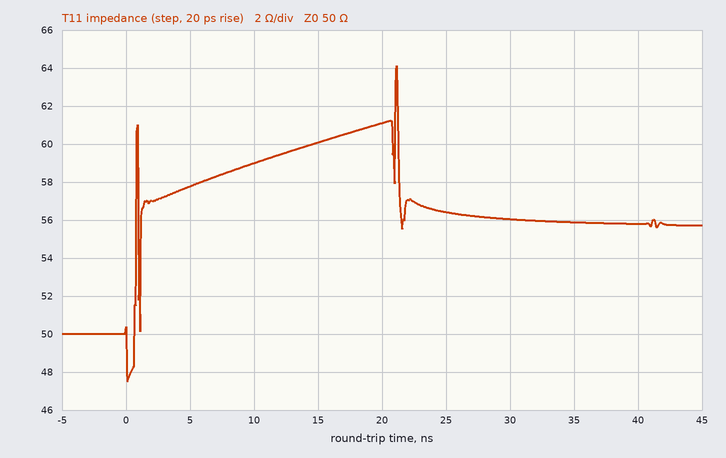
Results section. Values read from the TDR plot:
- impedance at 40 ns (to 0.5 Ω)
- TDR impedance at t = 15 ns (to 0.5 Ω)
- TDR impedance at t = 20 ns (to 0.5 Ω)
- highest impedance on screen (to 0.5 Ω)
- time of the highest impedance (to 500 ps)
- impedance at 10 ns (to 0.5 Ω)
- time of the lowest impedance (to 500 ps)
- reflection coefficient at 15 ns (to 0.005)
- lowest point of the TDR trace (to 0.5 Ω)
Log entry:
56.0 Ω
60.0 Ω
61.0 Ω
64.0 Ω
21.0 ns
59.0 Ω
0.0 ns
+0.090
47.5 Ω
